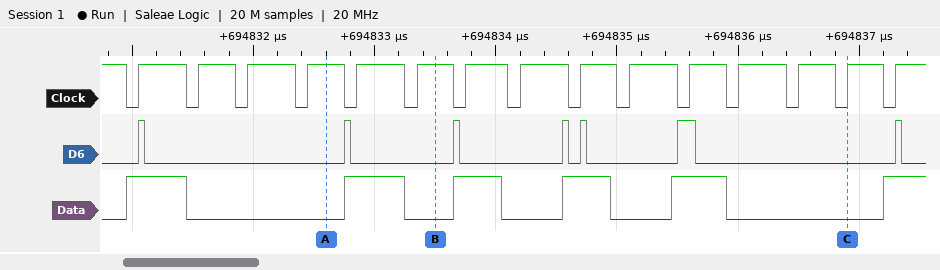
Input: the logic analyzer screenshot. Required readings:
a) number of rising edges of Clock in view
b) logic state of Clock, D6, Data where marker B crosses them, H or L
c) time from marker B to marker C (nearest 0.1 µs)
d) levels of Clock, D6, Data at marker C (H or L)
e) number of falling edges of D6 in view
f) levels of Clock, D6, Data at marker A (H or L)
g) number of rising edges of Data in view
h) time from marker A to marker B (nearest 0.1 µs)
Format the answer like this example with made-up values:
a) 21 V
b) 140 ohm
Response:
a) 15
b) Clock=H, D6=L, Data=L
c) 3.4 µs
d) Clock=H, D6=L, Data=L
e) 7
f) Clock=H, D6=L, Data=L
g) 6
h) 0.9 µs
